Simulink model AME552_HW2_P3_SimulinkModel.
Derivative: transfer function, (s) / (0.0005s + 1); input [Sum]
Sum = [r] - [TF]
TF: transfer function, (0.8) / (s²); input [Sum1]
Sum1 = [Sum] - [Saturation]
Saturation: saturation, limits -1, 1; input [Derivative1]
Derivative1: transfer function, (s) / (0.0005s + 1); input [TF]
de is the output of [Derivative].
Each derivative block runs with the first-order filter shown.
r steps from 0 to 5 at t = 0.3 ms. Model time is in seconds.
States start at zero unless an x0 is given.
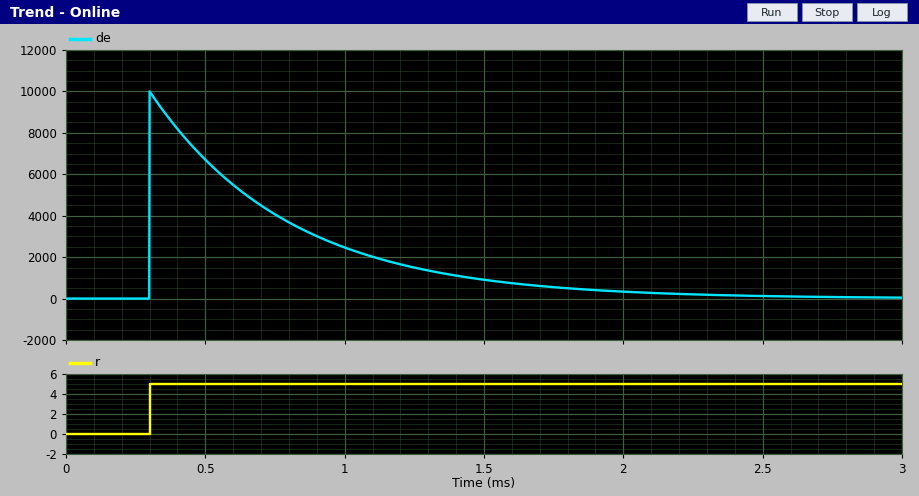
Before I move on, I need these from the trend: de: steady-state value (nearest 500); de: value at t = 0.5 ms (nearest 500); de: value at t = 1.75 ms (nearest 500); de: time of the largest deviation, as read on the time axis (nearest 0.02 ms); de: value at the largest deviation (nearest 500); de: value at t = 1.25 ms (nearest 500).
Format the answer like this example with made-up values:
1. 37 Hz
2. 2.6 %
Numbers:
1. 0
2. 6500
3. 500
4. 0.30 ms
5. 10000
6. 1500
